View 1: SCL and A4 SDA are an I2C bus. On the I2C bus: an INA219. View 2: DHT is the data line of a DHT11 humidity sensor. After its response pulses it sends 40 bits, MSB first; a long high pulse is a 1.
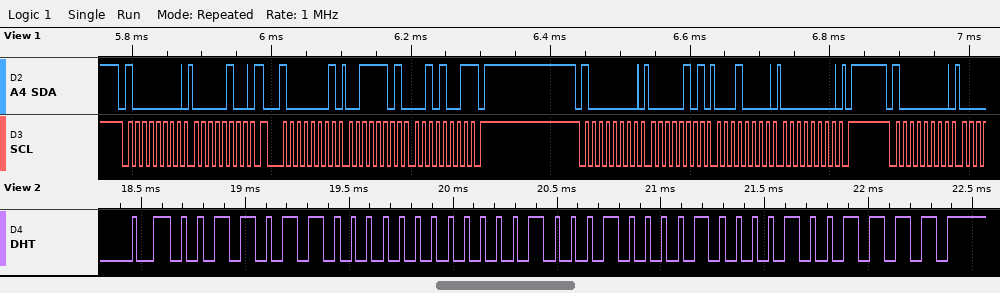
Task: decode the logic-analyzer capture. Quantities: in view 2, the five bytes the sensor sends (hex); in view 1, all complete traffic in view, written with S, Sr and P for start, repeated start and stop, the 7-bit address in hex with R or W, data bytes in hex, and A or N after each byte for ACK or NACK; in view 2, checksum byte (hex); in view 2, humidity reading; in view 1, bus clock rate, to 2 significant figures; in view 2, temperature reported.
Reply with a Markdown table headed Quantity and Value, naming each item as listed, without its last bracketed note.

| Quantity | Value |
|---|---|
| in view 2, the five bytes the sensor sends | 36 00 11 08 4F |
| in view 1, all complete traffic in view, written with S, Sr and P for start, repeated start and stop, the 7-bit address in hex with R or W, data bytes in hex, and A or N after each byte for ACK or NACK | S 40W A 04 A Sr 40R A 3D A 29 N P S 40W A 05 A 10 A 00 A P S 40W A |
| in view 2, checksum byte | 0x4F |
| in view 2, humidity reading | 54 % |
| in view 1, bus clock rate, to 2 significant figures | 100 kHz |
| in view 2, temperature reported | 17.8 °C |
